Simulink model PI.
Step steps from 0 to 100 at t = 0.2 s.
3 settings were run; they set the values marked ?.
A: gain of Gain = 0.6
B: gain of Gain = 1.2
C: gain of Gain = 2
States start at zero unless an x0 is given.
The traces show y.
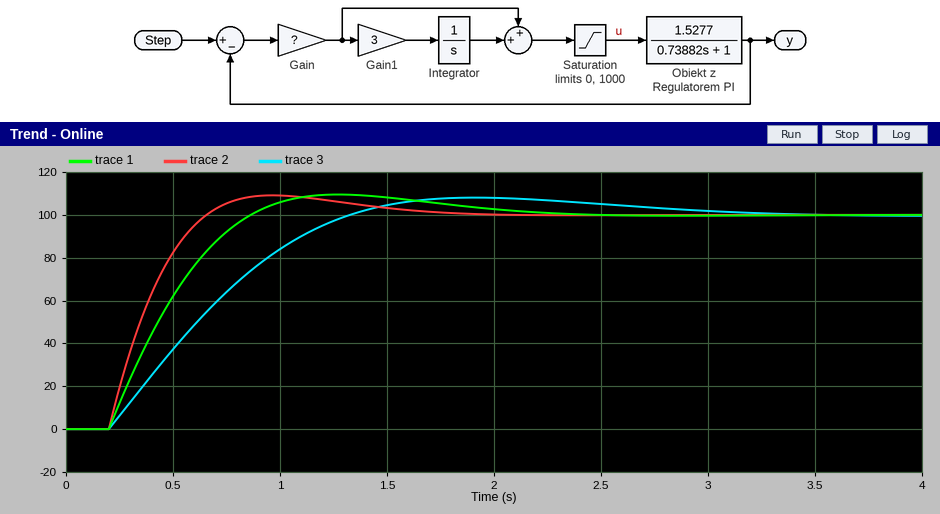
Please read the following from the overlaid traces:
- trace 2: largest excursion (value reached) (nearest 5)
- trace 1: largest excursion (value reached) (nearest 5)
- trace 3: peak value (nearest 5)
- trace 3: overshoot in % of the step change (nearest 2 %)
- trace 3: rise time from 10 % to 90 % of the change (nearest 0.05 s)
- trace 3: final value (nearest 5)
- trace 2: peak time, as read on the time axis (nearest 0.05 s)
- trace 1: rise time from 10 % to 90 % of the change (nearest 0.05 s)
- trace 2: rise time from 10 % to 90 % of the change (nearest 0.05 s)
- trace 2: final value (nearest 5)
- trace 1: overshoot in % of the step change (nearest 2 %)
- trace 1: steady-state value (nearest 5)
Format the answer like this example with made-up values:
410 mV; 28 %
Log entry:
110; 110; 110; 8 %; 0.80 s; 100; 0.95 s; 0.50 s; 0.35 s; 100; 10 %; 100
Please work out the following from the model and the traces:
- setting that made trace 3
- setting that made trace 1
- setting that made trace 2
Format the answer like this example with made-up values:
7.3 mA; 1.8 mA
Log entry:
A; B; C
